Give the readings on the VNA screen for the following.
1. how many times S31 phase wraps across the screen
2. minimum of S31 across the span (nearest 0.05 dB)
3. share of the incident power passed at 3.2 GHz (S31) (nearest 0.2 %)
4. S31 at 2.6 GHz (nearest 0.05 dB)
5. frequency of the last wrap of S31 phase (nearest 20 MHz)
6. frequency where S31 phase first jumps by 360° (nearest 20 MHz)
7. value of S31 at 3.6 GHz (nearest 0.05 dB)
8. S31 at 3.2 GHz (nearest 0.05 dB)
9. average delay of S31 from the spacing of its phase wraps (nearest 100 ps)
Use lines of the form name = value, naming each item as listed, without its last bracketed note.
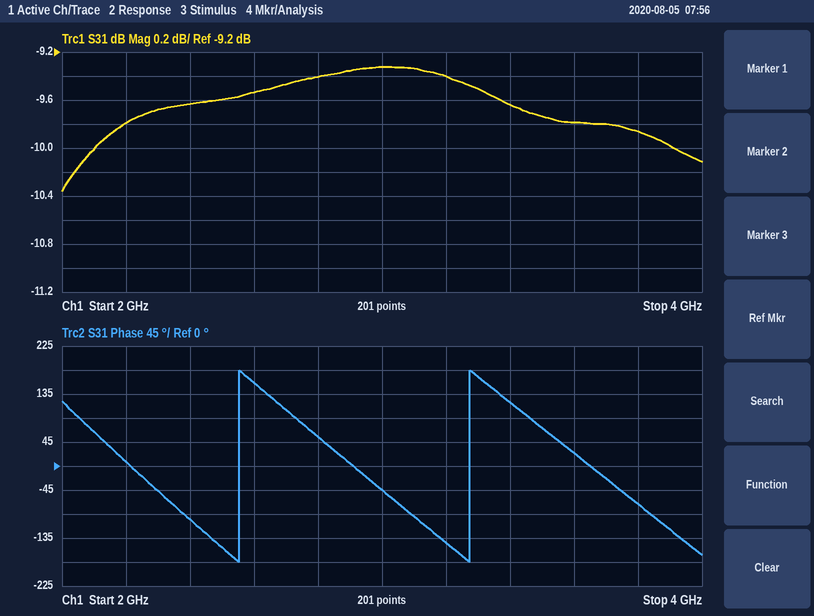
how many times S31 phase wraps across the screen = 2
minimum of S31 across the span = -10.35 dB
share of the incident power passed at 3.2 GHz (S31) = 11.4 %
S31 at 2.6 GHz = -9.55 dB
frequency of the last wrap of S31 phase = 3.28 GHz
frequency where S31 phase first jumps by 360° = 2.56 GHz
value of S31 at 3.6 GHz = -9.80 dB
S31 at 3.2 GHz = -9.40 dB
average delay of S31 from the spacing of its phase wraps = 1.4 ns
